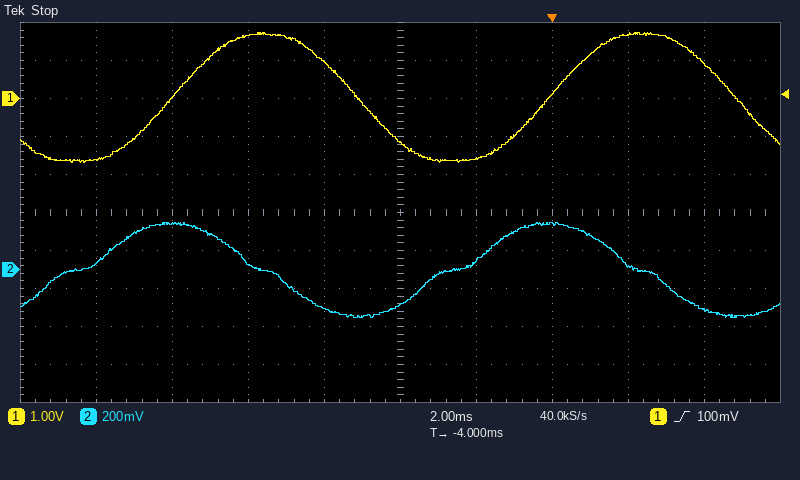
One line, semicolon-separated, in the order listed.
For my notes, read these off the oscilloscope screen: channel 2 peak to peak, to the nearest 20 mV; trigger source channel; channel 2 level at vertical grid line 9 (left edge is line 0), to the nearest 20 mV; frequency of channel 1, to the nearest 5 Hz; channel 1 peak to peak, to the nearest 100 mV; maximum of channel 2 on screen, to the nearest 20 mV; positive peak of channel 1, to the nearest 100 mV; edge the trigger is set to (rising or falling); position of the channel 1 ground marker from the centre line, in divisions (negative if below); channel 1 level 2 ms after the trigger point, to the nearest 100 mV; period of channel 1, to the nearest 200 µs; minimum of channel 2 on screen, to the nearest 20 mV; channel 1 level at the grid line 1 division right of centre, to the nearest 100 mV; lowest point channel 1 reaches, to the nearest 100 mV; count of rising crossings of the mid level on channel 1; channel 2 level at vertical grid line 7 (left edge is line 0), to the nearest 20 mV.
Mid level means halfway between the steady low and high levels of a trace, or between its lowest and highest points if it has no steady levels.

500 mV; channel 1; -220 mV; 100 Hz; 3.4 V; 240 mV; 1.7 V; rising; +3.0 div; 1.7 V; 10.0 ms; -260 mV; -1.6 V; -1.7 V; 2; 240 mV
